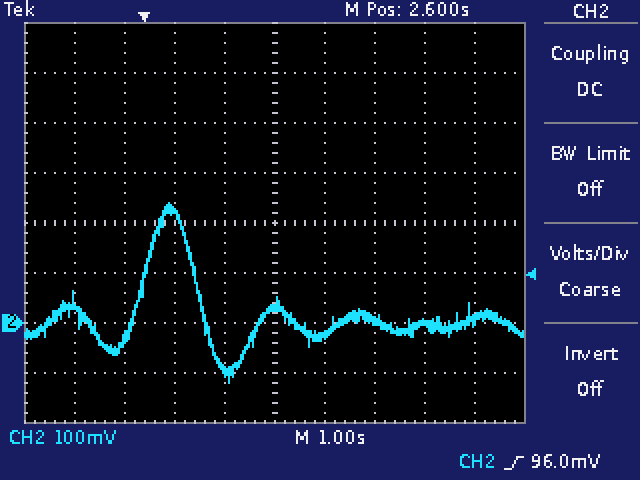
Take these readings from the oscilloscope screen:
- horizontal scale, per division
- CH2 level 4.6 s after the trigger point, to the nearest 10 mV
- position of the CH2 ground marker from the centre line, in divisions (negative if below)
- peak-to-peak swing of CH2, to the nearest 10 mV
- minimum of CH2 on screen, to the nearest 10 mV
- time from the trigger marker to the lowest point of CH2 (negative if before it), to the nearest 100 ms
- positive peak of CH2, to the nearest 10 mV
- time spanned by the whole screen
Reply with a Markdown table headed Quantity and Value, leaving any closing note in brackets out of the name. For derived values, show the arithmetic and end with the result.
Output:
| Quantity | Value |
|---|---|
| horizontal scale, per division | 1 s |
| CH2 level 4.6 s after the trigger point, to the nearest 10 mV | 10 mV |
| position of the CH2 ground marker from the centre line, in divisions | -2.0 div |
| peak-to-peak swing of CH2, to the nearest 10 mV | 240 mV − (-120 mV) = 360 mV |
| minimum of CH2 on screen, to the nearest 10 mV | -120 mV |
| time from the trigger marker to the lowest point of CH2 (negative if before it), to the nearest 100 ms | +1.7 s |
| positive peak of CH2, to the nearest 10 mV | 240 mV |
| time spanned by the whole screen | 10 s |
